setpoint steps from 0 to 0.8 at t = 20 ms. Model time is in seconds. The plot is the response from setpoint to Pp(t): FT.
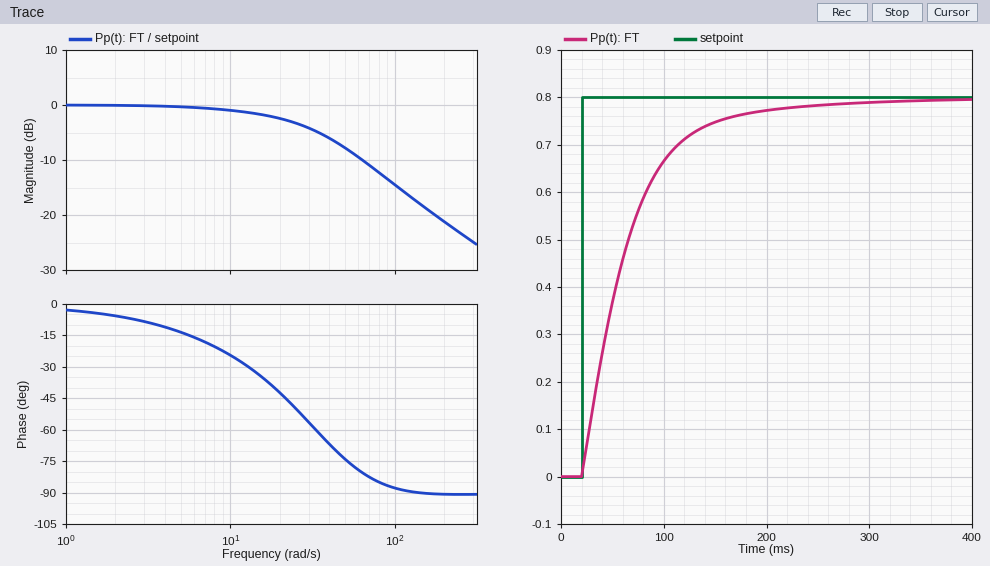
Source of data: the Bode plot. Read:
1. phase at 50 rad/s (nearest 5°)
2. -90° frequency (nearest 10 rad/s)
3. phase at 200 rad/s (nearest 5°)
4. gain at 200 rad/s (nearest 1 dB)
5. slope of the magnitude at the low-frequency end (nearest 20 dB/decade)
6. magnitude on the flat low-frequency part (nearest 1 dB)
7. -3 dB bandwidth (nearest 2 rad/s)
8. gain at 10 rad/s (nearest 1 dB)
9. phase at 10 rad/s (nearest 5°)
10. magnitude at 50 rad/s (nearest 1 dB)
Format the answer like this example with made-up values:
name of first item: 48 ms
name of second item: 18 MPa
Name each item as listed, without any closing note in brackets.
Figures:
phase at 50 rad/s: -75°
-90° frequency: 140 rad/s
phase at 200 rad/s: -90°
gain at 200 rad/s: -21 dB
slope of the magnitude at the low-frequency end: 0 dB/decade
magnitude on the flat low-frequency part: 0 dB
-3 dB bandwidth: 24 rad/s
gain at 10 rad/s: -1 dB
phase at 10 rad/s: -25°
magnitude at 50 rad/s: -8 dB
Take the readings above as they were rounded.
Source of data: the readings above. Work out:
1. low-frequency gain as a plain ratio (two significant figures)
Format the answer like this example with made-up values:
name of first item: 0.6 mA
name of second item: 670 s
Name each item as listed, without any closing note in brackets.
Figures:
low-frequency gain as a plain ratio: 1.0
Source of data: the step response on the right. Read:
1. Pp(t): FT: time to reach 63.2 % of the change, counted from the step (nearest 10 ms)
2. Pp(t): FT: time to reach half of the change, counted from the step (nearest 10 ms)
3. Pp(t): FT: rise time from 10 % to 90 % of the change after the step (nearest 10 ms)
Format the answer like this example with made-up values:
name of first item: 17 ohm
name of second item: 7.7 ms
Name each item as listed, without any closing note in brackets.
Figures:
Pp(t): FT: time to reach 63.2 % of the change, counted from the step: 50 ms
Pp(t): FT: time to reach half of the change, counted from the step: 30 ms
Pp(t): FT: rise time from 10 % to 90 % of the change after the step: 100 ms
